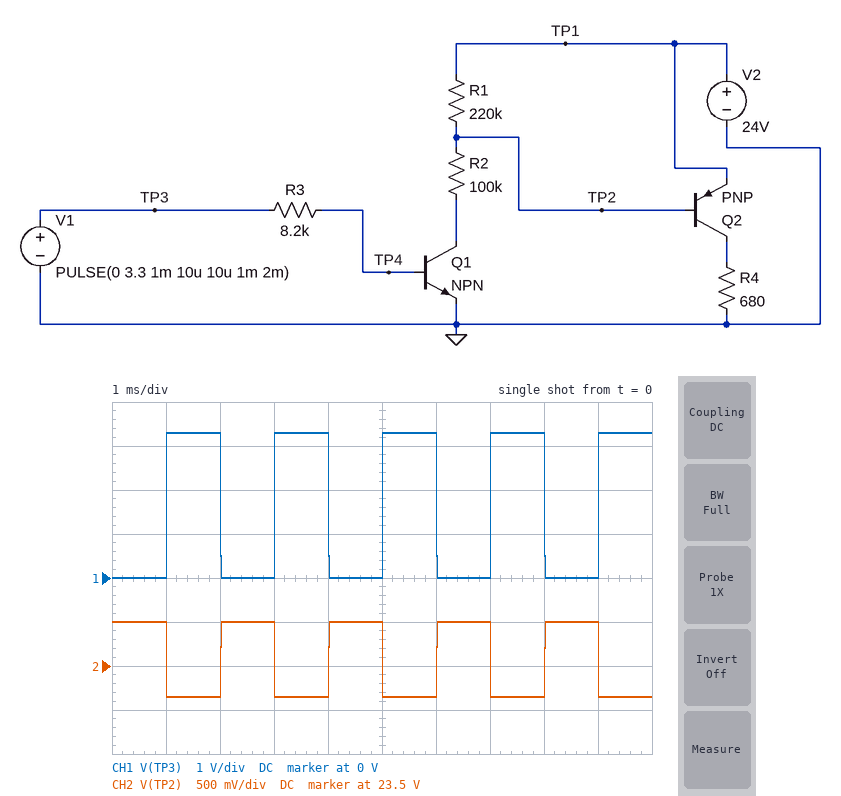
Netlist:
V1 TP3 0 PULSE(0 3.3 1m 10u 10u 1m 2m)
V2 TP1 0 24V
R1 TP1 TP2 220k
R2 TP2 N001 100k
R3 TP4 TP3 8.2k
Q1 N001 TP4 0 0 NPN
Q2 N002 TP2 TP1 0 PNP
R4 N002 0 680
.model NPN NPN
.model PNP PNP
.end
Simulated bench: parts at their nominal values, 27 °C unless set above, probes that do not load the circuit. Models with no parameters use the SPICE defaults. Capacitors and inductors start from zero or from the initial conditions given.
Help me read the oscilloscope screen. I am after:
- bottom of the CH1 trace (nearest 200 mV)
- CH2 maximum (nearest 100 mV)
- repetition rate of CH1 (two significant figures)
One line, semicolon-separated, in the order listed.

0 V; 24.0 V; 500 Hz
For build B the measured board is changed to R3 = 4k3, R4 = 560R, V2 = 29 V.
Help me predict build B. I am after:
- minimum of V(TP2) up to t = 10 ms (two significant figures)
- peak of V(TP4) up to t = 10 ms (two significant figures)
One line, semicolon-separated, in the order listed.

28 V; 780 mV
